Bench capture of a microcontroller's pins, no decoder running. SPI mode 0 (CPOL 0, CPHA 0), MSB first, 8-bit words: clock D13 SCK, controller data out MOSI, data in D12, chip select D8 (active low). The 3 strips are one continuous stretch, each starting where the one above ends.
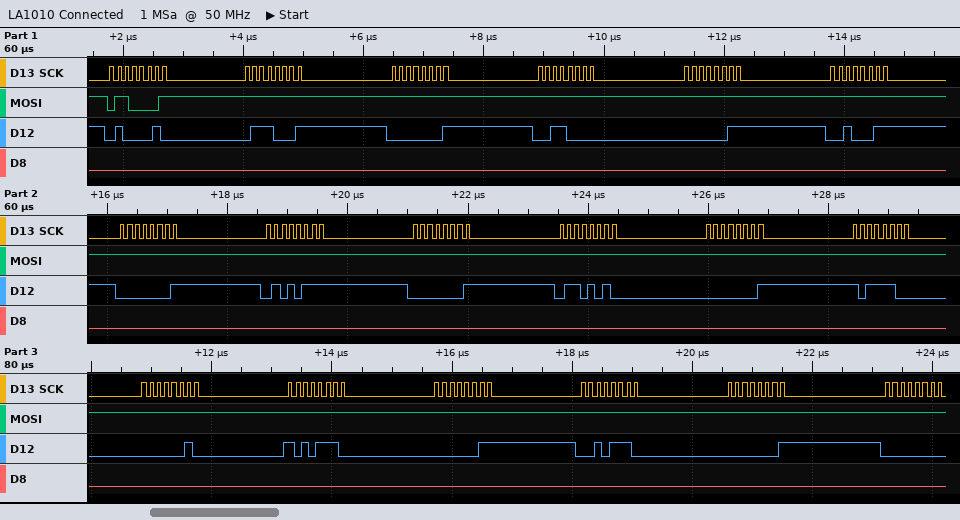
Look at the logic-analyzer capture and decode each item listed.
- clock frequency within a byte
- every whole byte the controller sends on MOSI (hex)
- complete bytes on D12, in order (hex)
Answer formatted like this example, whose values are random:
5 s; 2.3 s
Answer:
8 MHz; 0x61 0xFF 0xFF 0xFF 0xFF 0xFF 0xFF 0xFF 0xFF 0xFF 0xFF 0xFF 0xFF 0xFF 0xFF 0xFF 0xFF 0xFF; 0x42 0x71 0x01 0x30 0x03 0x23 0x01 0x57 0x01 0x6A 0x01 0xBC 0x02 0xAE 0x03 0x2E 0x01 0x00
